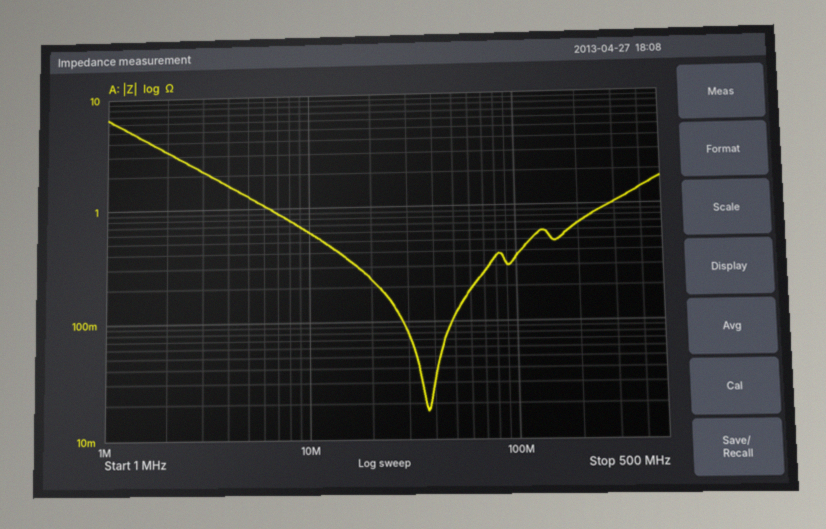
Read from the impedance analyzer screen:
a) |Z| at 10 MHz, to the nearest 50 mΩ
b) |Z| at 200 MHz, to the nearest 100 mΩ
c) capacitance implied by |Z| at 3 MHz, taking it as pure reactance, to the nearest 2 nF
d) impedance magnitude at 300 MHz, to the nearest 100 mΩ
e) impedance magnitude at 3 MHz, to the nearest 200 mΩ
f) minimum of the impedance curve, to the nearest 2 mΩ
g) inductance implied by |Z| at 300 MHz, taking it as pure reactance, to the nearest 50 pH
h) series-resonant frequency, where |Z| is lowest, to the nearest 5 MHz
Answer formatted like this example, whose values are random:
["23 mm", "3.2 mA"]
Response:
["600 mΩ", "700 mΩ", "24 nF", "1.0 Ω", "2.2 Ω", "18 mΩ", "550 pH", "35 MHz"]
